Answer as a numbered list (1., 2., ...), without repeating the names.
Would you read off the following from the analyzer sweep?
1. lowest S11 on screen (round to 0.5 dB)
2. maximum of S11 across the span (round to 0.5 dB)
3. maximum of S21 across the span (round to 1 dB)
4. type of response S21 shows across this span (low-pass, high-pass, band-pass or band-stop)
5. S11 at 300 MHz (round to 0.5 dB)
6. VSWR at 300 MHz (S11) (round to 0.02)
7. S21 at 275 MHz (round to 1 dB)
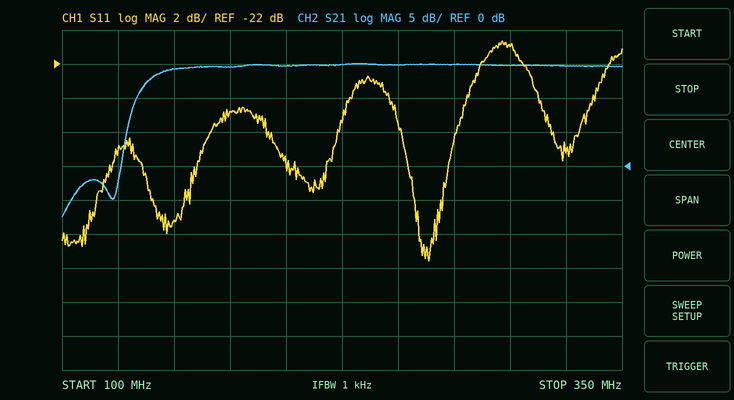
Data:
1. -33.5 dB
2. -20.5 dB
3. 15 dB
4. high-pass
5. -21.0 dB
6. 1.20
7. 15 dB
